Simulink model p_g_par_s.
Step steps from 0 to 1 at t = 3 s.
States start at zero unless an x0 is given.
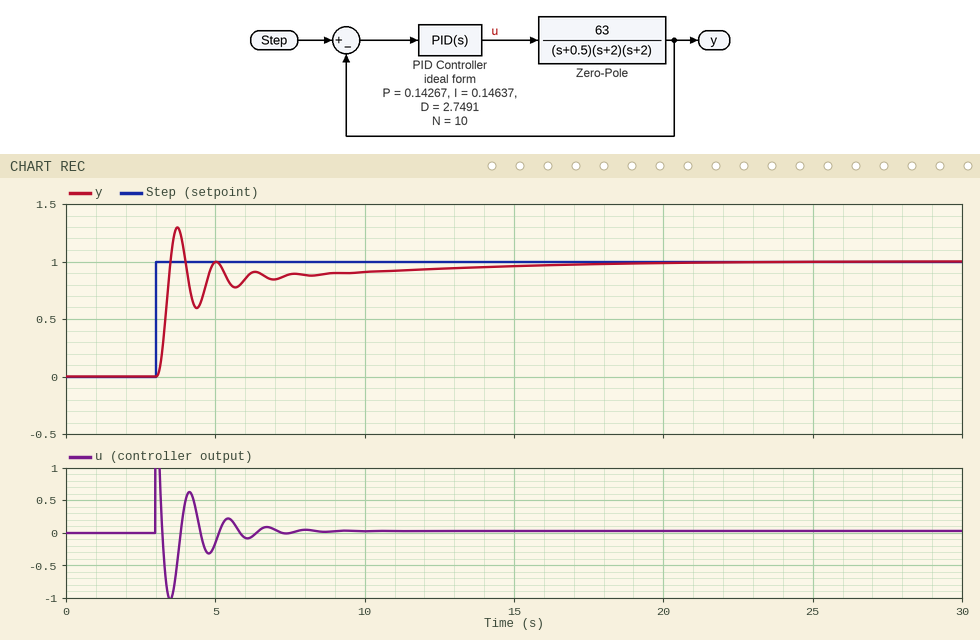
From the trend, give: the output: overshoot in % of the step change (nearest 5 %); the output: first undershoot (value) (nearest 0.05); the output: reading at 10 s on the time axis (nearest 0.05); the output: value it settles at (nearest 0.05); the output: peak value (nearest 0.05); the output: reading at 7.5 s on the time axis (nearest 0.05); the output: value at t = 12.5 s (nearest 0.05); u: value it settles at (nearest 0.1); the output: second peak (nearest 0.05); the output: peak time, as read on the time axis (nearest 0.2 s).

30 %
0.60
0.90
1.00
1.30
0.90
0.95
0.0
1.00
3.8 s
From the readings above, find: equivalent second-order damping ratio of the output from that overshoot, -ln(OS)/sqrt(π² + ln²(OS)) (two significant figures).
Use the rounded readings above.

0.36
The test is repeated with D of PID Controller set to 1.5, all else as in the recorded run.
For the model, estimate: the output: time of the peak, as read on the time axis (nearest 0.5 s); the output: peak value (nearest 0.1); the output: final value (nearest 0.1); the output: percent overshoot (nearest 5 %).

4.0 s
1.1
1.0
10 %
